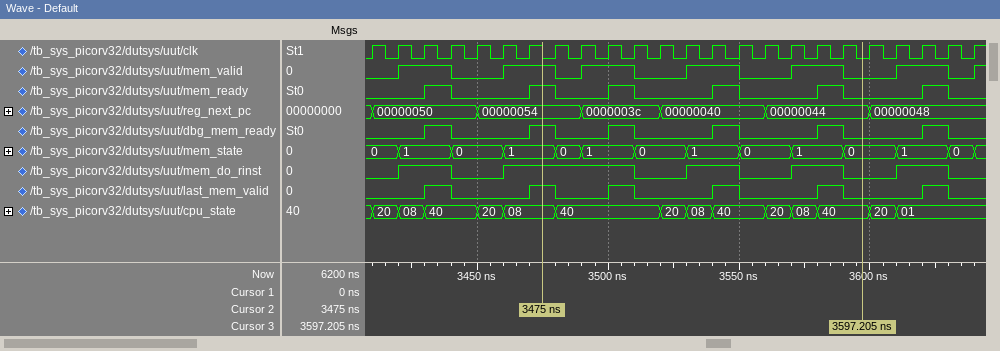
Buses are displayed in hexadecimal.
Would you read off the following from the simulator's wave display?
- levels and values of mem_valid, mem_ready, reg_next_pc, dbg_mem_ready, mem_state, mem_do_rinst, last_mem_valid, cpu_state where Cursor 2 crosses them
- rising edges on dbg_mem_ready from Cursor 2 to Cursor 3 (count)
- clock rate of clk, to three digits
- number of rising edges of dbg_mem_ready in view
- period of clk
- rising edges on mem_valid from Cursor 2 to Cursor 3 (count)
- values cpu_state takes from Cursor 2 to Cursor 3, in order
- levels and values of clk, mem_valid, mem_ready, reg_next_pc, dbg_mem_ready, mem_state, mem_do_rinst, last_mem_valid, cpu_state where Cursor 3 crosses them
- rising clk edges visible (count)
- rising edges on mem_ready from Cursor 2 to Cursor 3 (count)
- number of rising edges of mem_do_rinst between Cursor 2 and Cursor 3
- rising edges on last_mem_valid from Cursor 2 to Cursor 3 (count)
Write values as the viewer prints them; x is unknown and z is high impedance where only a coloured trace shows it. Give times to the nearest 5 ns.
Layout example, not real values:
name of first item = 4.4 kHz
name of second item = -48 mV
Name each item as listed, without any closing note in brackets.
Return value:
levels and values of mem_valid, mem_ready, reg_next_pc, dbg_mem_ready, mem_state, mem_do_rinst, last_mem_valid, cpu_state where Cursor 2 crosses them = mem_valid=1, mem_ready=1, reg_next_pc=00000054, dbg_mem_ready=1, mem_state=1, mem_do_rinst=1, last_mem_valid=1, cpu_state=08
rising edges on dbg_mem_ready from Cursor 2 to Cursor 3 = 3
clock rate of clk, to three digits = 100 MHz
number of rising edges of dbg_mem_ready in view = 6
period of clk = 10 ns
rising edges on mem_valid from Cursor 2 to Cursor 3 = 3
values cpu_state takes from Cursor 2 to Cursor 3, in order = 08, 40, 20, 08, 40, 20, 08, 40
levels and values of clk, mem_valid, mem_ready, reg_next_pc, dbg_mem_ready, mem_state, mem_do_rinst, last_mem_valid, cpu_state where Cursor 3 crosses them = clk=0, mem_valid=0, mem_ready=0, reg_next_pc=00000044, dbg_mem_ready=0, mem_state=0, mem_do_rinst=0, last_mem_valid=0, cpu_state=40
rising clk edges visible = 24
rising edges on mem_ready from Cursor 2 to Cursor 3 = 3
number of rising edges of mem_do_rinst between Cursor 2 and Cursor 3 = 2
rising edges on last_mem_valid from Cursor 2 to Cursor 3 = 3
